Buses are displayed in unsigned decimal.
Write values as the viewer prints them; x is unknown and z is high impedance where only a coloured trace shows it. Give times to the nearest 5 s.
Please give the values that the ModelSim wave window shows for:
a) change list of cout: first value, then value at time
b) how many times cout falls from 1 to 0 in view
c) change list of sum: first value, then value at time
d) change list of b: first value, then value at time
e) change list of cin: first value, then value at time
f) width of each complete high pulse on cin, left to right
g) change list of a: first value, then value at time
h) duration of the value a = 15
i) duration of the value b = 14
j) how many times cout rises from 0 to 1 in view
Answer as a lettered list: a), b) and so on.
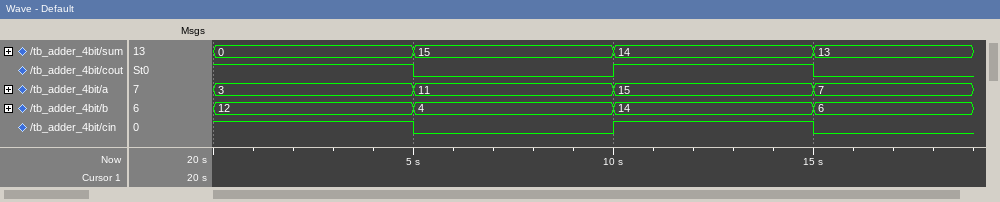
a) 1, 0 at 5 s, 1 at 10 s, 0 at 15 s
b) 2
c) 0, 15 at 5 s, 14 at 10 s, 13 at 15 s
d) 12, 4 at 5 s, 14 at 10 s, 6 at 15 s
e) 1, 0 at 5 s, 1 at 10 s, 0 at 15 s
f) 5 s
g) 3, 11 at 5 s, 15 at 10 s, 7 at 15 s
h) 5 s
i) 5 s
j) 1
